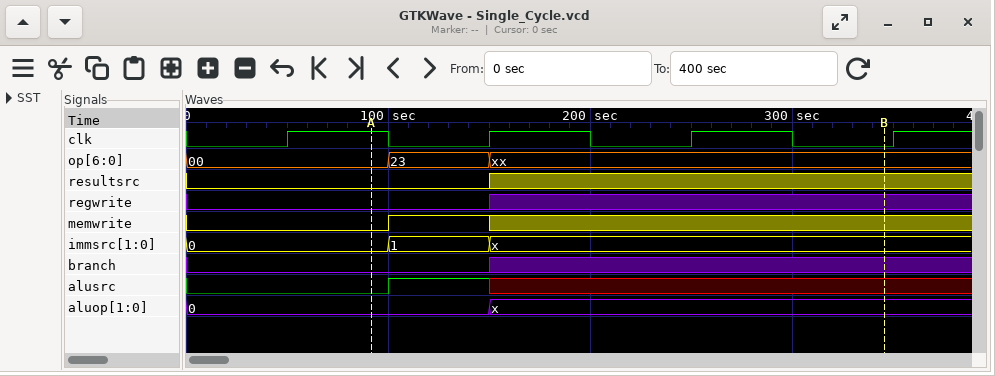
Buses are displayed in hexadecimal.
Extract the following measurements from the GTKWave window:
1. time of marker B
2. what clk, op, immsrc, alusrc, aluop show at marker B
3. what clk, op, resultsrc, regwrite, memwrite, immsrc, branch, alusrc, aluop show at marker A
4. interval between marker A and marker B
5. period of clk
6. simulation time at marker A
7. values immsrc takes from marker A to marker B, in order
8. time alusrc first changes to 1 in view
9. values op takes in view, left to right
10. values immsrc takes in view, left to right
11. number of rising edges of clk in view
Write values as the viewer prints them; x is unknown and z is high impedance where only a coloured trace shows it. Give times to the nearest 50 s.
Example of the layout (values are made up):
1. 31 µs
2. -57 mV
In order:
1. 350 s
2. clk=0, op=xx, immsrc=x, alusrc=x, aluop=x
3. clk=1, op=00, resultsrc=0, regwrite=0, memwrite=0, immsrc=0, branch=0, alusrc=0, aluop=0
4. 250 s
5. 100 s
6. 100 s
7. 0, 1, x
8. 100 s
9. 00, 23, xx
10. 0, 1, x
11. 4
